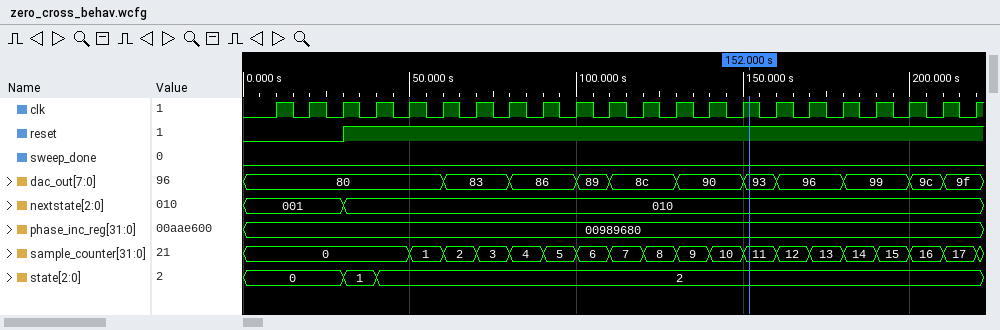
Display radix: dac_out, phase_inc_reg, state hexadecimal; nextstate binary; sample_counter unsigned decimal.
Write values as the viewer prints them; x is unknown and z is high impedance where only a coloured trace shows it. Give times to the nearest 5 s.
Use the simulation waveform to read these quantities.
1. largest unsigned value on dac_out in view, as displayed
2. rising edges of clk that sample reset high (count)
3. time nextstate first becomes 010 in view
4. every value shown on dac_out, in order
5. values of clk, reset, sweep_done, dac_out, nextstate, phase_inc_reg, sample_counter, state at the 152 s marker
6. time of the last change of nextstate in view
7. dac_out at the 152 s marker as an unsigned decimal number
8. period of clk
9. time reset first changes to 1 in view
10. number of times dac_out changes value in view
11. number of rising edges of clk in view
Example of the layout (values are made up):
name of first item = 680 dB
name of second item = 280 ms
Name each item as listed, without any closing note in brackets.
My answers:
largest unsigned value on dac_out in view, as displayed = 9f
rising edges of clk that sample reset high = 19
time nextstate first becomes 010 in view = 30 s
every value shown on dac_out, in order = 80, 83, 86, 89, 8c, 90, 93, 96, 99, 9c, 9f
values of clk, reset, sweep_done, dac_out, nextstate, phase_inc_reg, sample_counter, state at the 152 s marker = clk=1, reset=1, sweep_done=0, dac_out=93, nextstate=010, phase_inc_reg=00989680, sample_counter=11, state=2
time of the last change of nextstate in view = 30 s
dac_out at the 152 s marker as an unsigned decimal number = 147
period of clk = 10 s
time reset first changes to 1 in view = 30 s
number of times dac_out changes value in view = 10
number of rising edges of clk in view = 22
